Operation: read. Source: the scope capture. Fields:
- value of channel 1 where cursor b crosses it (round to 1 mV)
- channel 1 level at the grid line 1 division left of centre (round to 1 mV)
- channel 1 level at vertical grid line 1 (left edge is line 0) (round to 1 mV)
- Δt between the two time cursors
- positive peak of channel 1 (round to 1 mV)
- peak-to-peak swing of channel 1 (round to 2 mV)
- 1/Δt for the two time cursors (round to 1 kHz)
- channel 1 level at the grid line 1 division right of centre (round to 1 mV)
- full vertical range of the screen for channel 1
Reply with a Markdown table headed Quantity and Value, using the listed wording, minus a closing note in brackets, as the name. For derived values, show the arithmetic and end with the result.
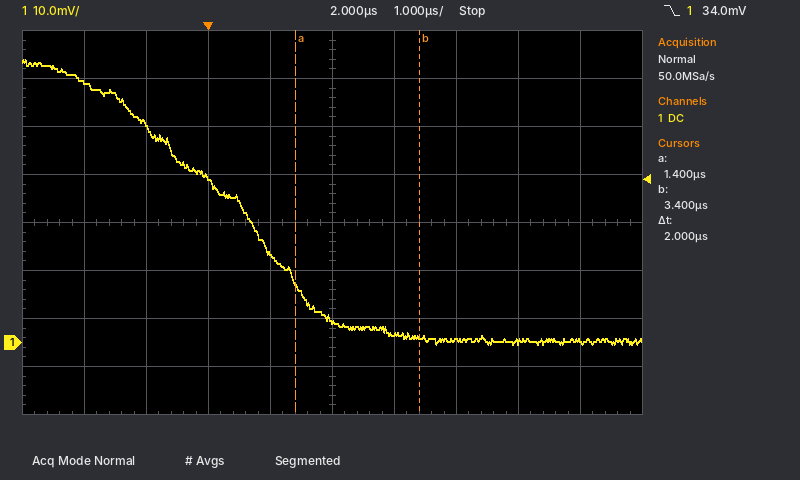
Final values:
| Quantity | Value |
|---|---|
| value of channel 1 where cursor b crosses it | 1 mV |
| channel 1 level at the grid line 1 division left of centre | 18 mV |
| channel 1 level at vertical grid line 1 (left edge is line 0) | 54 mV |
| Δt between the two time cursors | 2 µs |
| positive peak of channel 1 | 59 mV |
| peak-to-peak swing of channel 1 | 60 mV |
| 1/Δt for the two time cursors | 1 / 2 µs ≈ 500 kHz |
| channel 1 level at the grid line 1 division right of centre | 2 mV |
| full vertical range of the screen for channel 1 | 80 mV |
